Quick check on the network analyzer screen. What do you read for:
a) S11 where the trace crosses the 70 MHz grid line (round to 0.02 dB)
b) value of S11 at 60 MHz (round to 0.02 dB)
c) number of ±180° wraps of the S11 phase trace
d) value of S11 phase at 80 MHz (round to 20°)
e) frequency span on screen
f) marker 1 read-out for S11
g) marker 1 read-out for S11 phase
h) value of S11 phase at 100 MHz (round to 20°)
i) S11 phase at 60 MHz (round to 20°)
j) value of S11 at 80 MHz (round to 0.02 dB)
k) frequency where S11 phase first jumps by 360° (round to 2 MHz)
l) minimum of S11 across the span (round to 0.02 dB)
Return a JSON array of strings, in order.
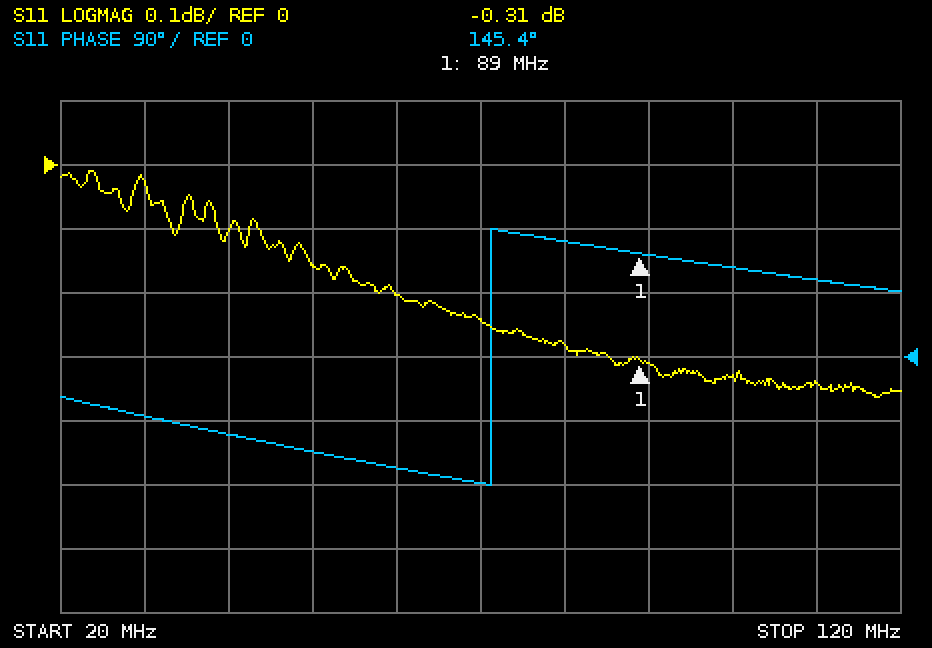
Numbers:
["-0.24 dB", "-0.20 dB", "1", "160°", "100 MHz", "-0.31 dB", "145.4°", "120°", "-160°", "-0.28 dB", "72 MHz", "-0.36 dB"]
